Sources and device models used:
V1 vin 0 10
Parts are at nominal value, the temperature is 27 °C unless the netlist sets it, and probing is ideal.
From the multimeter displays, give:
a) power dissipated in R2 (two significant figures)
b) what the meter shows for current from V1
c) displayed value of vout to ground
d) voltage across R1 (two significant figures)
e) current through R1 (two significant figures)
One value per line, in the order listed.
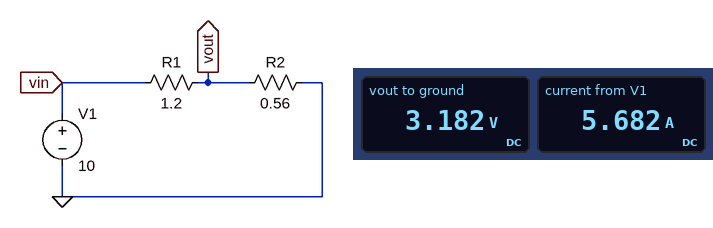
18 W
5.682 A
3.182 V
6.8 V
5.7 A
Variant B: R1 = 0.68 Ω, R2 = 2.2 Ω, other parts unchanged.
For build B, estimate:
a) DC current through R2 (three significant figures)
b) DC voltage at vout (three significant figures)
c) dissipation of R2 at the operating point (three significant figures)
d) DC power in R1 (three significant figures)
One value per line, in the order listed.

3.47 A
7.64 V
26.5 W
8.20 W
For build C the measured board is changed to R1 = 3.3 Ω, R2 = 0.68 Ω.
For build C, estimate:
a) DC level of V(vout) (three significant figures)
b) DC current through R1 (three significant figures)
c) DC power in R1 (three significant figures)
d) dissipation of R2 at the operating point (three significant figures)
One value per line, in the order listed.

1.71 V
2.51 A
20.8 W
4.29 W
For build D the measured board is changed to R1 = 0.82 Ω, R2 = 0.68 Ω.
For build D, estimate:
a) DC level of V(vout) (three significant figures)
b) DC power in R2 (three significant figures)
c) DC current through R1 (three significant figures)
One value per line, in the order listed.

4.53 V
30.2 W
6.67 A
